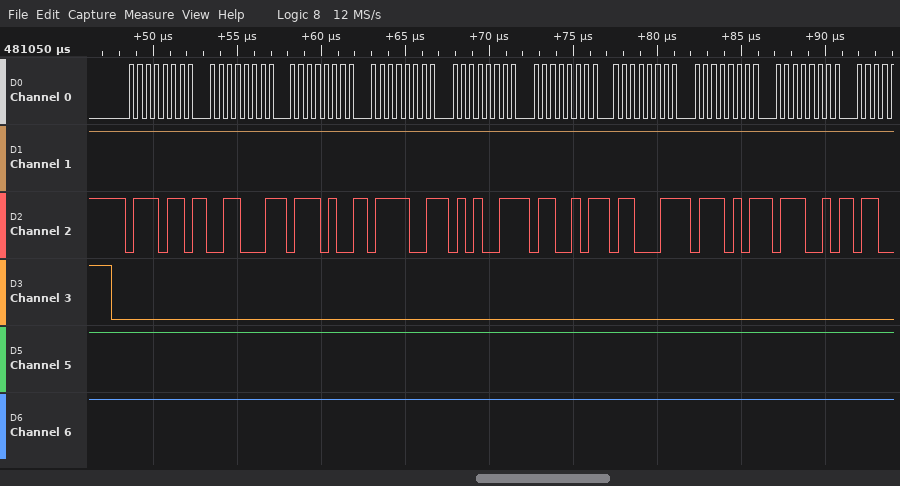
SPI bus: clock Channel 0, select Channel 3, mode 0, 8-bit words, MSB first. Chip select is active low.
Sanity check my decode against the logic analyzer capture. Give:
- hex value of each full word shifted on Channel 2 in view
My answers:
76, 31, 74, 79, 53, 65, 63, 75, 72
